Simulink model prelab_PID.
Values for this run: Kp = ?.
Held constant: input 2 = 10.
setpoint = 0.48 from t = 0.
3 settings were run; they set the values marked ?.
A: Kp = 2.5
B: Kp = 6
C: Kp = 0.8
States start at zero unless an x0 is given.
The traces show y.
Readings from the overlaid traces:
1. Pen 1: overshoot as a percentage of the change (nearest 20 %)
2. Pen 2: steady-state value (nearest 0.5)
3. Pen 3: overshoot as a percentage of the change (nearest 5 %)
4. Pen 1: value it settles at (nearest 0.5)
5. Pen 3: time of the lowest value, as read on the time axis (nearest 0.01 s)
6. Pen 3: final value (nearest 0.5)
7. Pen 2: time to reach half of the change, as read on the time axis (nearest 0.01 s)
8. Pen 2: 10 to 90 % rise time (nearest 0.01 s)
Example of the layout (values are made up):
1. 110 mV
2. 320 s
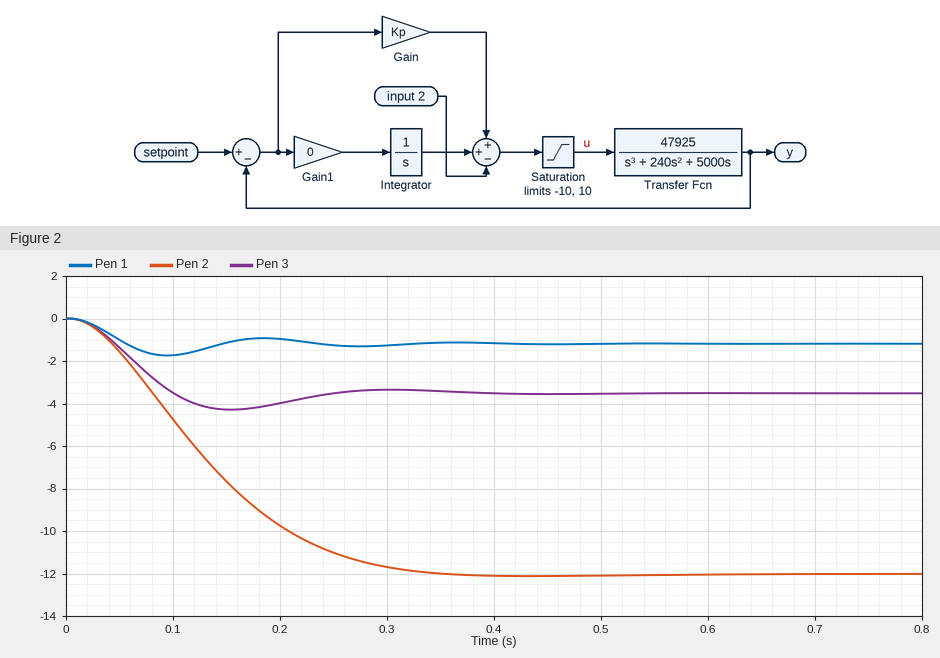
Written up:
1. 40 %
2. -12.0
3. 20 %
4. -1.0
5. 0.15 s
6. -3.5
7. 0.12 s
8. 0.20 s
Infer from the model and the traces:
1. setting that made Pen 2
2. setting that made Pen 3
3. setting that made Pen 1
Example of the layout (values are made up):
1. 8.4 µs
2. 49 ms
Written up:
1. C
2. A
3. B
